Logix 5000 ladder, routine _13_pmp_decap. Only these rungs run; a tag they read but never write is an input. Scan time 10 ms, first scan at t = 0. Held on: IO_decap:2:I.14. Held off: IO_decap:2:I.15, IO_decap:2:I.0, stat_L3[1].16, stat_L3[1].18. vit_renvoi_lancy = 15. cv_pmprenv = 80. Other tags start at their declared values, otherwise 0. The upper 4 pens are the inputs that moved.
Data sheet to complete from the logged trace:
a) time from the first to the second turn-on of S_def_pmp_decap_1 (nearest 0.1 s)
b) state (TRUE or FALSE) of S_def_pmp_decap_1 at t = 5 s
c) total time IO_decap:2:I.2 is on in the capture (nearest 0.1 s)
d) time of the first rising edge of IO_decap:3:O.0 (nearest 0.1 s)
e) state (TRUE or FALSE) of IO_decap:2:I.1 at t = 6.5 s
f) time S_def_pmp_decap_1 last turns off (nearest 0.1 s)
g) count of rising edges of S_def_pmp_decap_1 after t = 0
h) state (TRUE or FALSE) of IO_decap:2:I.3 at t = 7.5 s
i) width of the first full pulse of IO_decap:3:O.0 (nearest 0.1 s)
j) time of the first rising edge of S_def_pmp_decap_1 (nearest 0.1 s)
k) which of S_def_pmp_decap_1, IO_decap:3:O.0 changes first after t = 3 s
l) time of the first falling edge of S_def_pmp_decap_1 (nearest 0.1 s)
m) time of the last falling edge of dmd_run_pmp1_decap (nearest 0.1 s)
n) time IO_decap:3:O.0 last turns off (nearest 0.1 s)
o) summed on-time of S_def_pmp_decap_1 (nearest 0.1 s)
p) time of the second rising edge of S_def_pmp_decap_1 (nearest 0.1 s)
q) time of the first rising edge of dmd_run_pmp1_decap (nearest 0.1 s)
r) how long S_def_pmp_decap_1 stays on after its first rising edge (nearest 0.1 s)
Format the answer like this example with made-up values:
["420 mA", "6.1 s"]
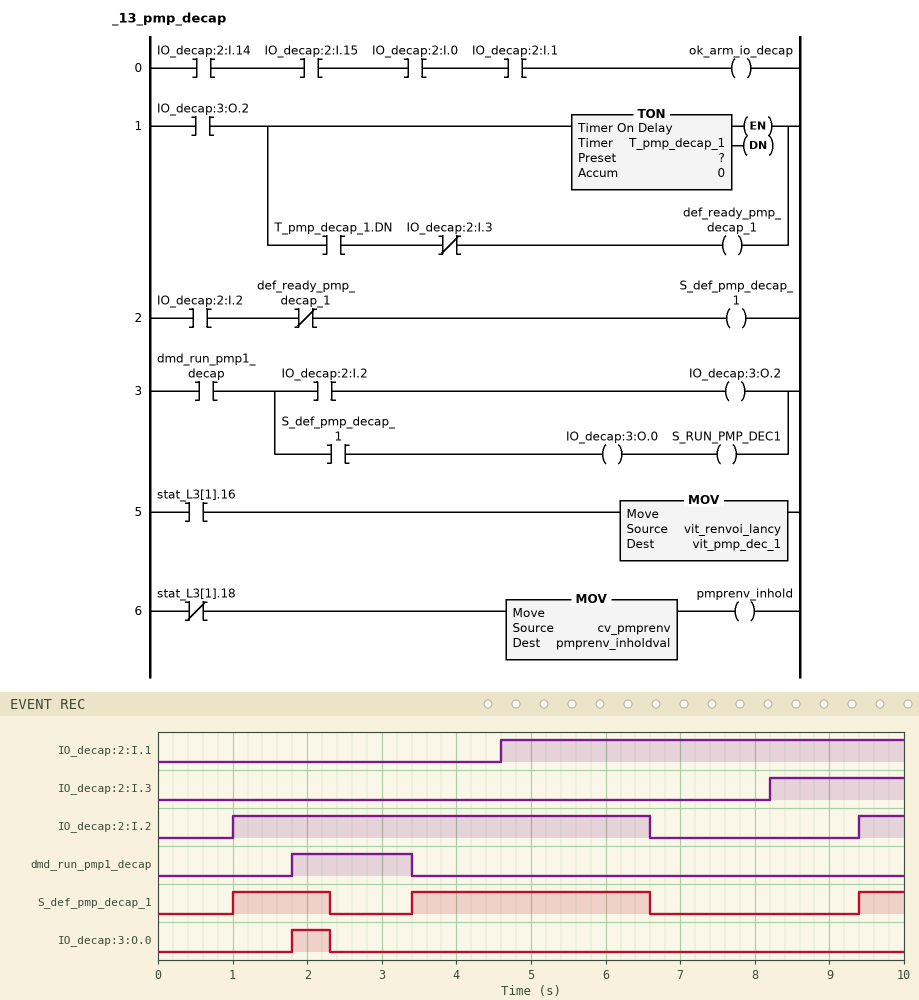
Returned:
["2.4 s", "TRUE", "6.2 s", "1.8 s", "TRUE", "6.6 s", "3", "FALSE", "0.5 s", "1.0 s", "S_def_pmp_decap_1", "2.3 s", "3.4 s", "2.3 s", "5.1 s", "3.4 s", "1.8 s", "1.3 s"]
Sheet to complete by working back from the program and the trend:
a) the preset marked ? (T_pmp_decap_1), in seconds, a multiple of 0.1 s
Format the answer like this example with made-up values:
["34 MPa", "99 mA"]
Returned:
["0.5 s"]
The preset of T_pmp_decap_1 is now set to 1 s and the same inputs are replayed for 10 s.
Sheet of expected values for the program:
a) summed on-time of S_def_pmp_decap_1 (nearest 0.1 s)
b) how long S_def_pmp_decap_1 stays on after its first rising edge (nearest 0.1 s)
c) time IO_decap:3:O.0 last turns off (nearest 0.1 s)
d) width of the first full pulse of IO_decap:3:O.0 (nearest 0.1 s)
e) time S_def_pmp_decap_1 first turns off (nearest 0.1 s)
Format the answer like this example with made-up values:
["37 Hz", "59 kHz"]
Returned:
["5.6 s", "1.8 s", "2.8 s", "1.0 s", "2.8 s"]
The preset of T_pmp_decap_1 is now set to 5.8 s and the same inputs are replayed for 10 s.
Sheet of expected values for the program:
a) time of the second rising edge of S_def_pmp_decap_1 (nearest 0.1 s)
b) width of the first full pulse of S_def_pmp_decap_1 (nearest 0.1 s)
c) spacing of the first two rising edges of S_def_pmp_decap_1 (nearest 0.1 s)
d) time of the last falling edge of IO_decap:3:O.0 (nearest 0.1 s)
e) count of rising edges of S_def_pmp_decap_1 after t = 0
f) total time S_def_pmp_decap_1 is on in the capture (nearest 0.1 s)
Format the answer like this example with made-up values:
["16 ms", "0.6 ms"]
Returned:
["9.4 s", "5.6 s", "8.4 s", "3.4 s", "2", "6.2 s"]
